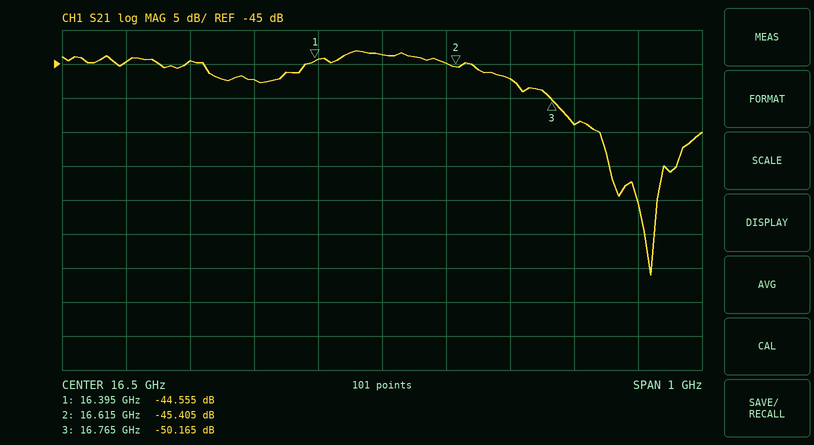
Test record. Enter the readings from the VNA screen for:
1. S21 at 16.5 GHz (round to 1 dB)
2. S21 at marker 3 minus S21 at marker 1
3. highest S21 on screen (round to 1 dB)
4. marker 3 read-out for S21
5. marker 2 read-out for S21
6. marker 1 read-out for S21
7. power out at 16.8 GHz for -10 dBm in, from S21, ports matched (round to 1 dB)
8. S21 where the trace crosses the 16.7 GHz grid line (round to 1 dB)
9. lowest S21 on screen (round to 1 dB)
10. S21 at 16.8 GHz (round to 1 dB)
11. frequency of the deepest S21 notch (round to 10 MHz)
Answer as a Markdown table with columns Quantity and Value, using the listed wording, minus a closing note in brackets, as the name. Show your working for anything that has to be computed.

| Quantity | Value |
|---|---|
| S21 at 16.5 GHz | -44 dB |
| S21 at marker 3 minus S21 at marker 1 | -50.165 − (-44.555) = -5.610 dB |
| highest S21 on screen | -43 dB |
| marker 3 read-out for S21 | -50.165 dB |
| marker 2 read-out for S21 | -45.405 dB |
| marker 1 read-out for S21 | -44.555 dB |
| power out at 16.8 GHz for -10 dBm in, from S21, ports matched | -10 dBm + (-54 dB) = -64 dBm |
| S21 where the trace crosses the 16.7 GHz grid line | -47 dB |
| lowest S21 on screen | -76 dB |
| S21 at 16.8 GHz | -54 dB |
| frequency of the deepest S21 notch | 16.92 GHz |
